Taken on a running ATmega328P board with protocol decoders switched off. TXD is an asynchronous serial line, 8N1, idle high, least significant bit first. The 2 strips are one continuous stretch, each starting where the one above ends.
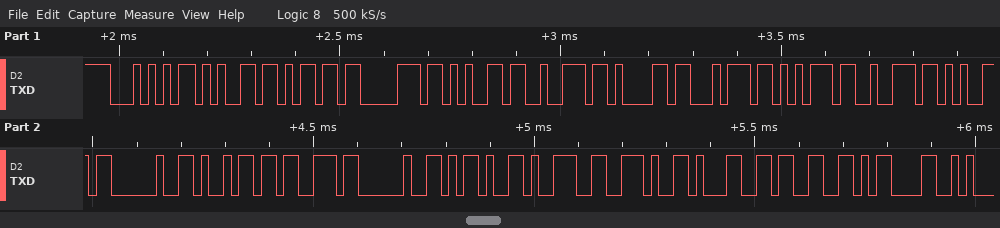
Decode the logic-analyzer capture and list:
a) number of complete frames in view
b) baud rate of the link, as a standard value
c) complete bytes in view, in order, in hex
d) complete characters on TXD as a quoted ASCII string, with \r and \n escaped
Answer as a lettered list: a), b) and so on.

a) 21
b) 57600 baud
c) 54 65 6D 70 65 72 61 74 75 72 65 20 69 73 20 2D 39 2E 31 33 0D
d) "Temperature is -9.13\r"
